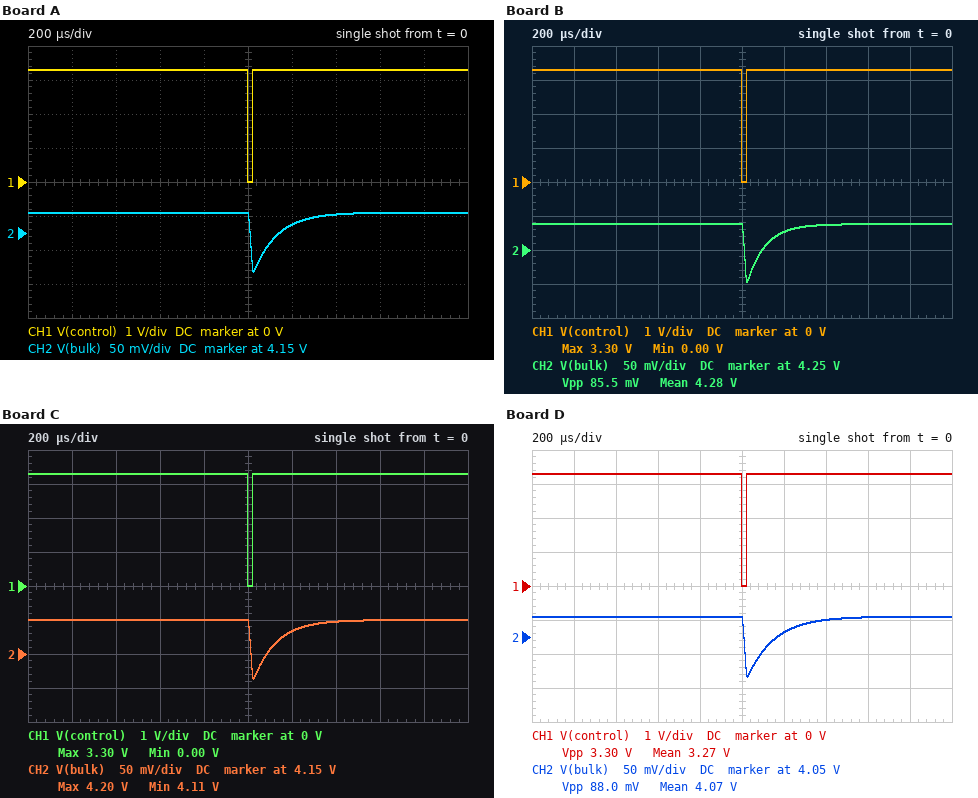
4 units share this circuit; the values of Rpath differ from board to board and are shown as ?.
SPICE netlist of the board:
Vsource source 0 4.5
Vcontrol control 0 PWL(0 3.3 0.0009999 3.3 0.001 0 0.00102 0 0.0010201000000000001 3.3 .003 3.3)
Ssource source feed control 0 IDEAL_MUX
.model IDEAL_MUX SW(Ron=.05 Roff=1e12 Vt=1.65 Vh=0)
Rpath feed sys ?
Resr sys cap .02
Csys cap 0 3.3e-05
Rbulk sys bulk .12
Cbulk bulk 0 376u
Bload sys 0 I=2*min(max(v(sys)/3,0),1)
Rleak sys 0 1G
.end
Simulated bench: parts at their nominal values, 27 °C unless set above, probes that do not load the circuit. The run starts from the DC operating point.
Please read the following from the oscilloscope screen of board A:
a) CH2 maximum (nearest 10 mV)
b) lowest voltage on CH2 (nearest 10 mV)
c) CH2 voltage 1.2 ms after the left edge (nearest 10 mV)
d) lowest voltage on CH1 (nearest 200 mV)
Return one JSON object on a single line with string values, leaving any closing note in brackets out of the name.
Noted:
{"CH2 maximum": "4.18 V", "lowest voltage on CH2": "4.09 V", "CH2 voltage 1.2 ms after the left edge": "4.16 V", "lowest voltage on CH1": "0 V"}
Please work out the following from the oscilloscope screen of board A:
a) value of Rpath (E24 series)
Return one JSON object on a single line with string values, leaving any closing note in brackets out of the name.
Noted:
{"value of Rpath": "0.11 Ω"}
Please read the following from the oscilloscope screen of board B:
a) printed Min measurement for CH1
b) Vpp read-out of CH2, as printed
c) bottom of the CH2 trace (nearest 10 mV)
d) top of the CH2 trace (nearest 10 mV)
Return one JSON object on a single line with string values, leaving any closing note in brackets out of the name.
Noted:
{"printed Min measurement for CH1": "0.00 V", "Vpp read-out of CH2, as printed": "85.5 mV", "bottom of the CH2 trace": "4.20 V", "top of the CH2 trace": "4.29 V"}
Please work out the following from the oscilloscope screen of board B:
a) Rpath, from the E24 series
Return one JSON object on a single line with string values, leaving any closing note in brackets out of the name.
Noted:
{"Rpath, from the E24 series": "0.056 Ω"}
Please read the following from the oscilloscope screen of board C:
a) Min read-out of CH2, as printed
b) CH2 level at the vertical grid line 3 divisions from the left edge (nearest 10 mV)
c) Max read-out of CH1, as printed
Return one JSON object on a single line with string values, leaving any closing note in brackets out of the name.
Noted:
{"Min read-out of CH2, as printed": "4.11 V", "CH2 level at the vertical grid line 3 divisions from the left edge": "4.20 V", "Max read-out of CH1, as printed": "3.30 V"}
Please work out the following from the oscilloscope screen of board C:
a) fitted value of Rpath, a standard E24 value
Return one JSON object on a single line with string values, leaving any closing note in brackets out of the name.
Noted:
{"fitted value of Rpath, a standard E24 value": "0.1 Ω"}
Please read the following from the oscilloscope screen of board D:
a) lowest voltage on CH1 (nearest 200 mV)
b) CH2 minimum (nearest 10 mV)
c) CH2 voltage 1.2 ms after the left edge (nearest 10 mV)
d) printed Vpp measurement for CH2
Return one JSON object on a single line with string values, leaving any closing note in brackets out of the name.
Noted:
{"lowest voltage on CH1": "0 V", "CH2 minimum": "3.99 V", "CH2 voltage 1.2 ms after the left edge": "4.06 V", "printed Vpp measurement for CH2": "88.0 mV"}
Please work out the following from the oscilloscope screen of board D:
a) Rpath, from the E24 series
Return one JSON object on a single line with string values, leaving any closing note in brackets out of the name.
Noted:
{"Rpath, from the E24 series": "0.16 Ω"}
